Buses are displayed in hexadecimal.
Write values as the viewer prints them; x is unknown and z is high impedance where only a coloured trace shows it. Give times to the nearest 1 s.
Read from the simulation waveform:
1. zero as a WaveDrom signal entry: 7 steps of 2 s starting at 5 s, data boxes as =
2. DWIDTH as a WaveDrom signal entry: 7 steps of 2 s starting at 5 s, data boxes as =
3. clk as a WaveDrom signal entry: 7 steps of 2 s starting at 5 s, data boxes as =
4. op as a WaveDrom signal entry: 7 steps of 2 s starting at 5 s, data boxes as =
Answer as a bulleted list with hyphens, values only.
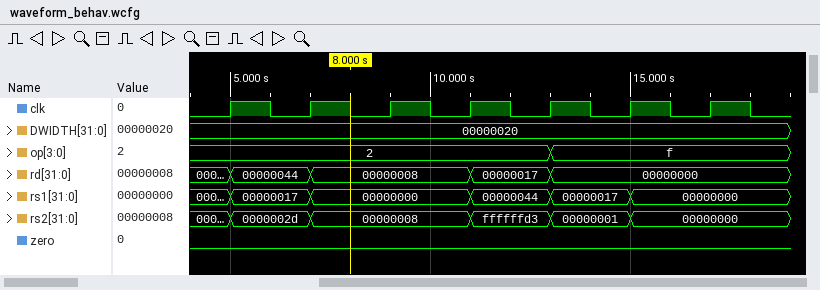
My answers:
- {name: 'zero', wave: '0......'}
- {name: 'DWIDTH', wave: '=......', data: '00000020'}
- {name: 'clk', wave: 'p......'}
- {name: 'op', wave: '=...=..', data: '2 f'}
